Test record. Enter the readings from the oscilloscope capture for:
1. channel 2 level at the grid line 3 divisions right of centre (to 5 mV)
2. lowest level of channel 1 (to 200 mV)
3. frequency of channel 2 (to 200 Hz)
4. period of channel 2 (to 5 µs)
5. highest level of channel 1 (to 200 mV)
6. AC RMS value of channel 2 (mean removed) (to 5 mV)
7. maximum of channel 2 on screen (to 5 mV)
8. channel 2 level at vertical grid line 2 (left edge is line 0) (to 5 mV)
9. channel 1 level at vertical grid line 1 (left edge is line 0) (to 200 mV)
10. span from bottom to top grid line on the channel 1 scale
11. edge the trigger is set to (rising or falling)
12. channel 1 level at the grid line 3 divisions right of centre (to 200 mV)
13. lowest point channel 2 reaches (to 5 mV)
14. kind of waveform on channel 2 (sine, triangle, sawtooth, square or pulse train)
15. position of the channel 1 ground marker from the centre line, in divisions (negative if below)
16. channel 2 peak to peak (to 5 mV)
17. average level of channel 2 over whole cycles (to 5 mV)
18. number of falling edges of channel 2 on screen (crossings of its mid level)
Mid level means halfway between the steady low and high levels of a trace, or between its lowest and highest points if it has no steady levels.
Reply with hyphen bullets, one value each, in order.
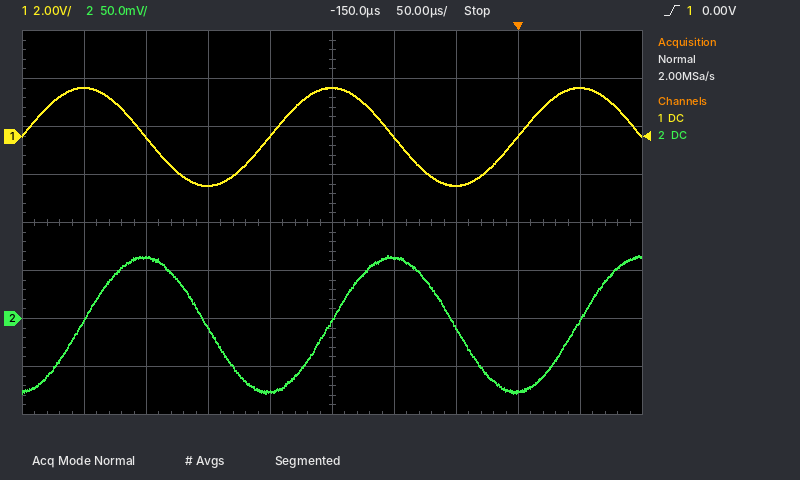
- -75 mV
- -2.0 V
- 5.0 kHz
- 200 µs
- 2.0 V
- 50 mV
- 65 mV
- 65 mV
- 2.0 V
- 16 V
- rising
- 0.0 V
- -80 mV
- sine
- +1.8 div
- 145 mV
- -5 mV
- 2
